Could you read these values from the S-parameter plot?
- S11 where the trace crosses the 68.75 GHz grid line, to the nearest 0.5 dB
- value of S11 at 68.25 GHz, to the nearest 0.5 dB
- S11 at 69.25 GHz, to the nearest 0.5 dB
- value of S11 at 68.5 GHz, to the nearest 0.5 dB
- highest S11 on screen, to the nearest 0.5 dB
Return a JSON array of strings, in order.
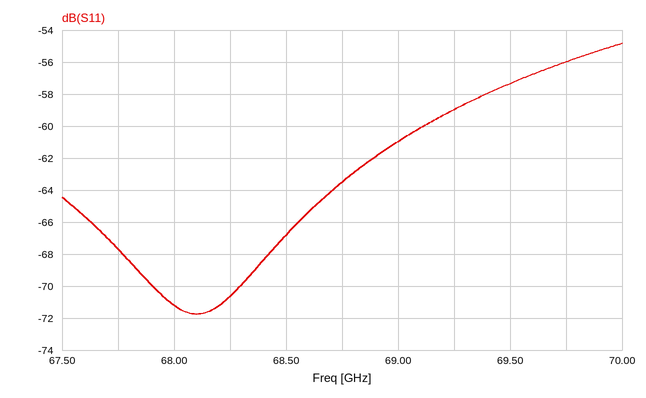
["-63.5 dB", "-70.5 dB", "-59.0 dB", "-67.0 dB", "-55.0 dB"]
